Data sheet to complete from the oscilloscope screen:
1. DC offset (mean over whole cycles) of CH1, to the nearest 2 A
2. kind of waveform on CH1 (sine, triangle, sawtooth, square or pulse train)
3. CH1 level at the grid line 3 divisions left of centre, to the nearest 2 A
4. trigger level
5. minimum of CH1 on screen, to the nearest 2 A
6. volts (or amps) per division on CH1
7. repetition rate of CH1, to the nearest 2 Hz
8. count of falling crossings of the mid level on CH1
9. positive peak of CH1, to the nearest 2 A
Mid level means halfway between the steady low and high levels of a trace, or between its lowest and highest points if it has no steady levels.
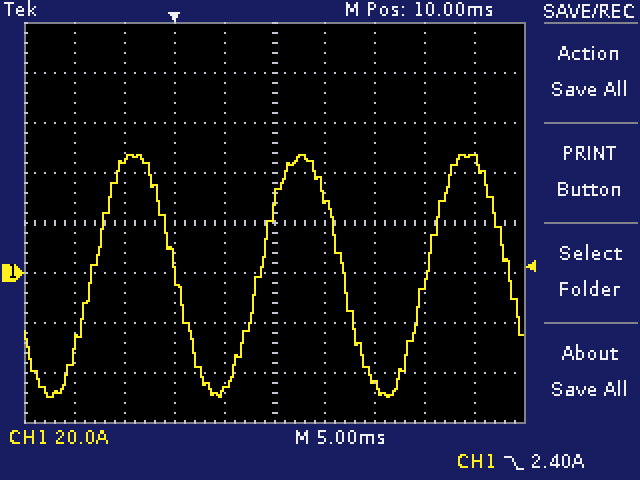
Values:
0 A
sine
46 A
2.40 A
-50 A
20 A
60 Hz
3
48 A
